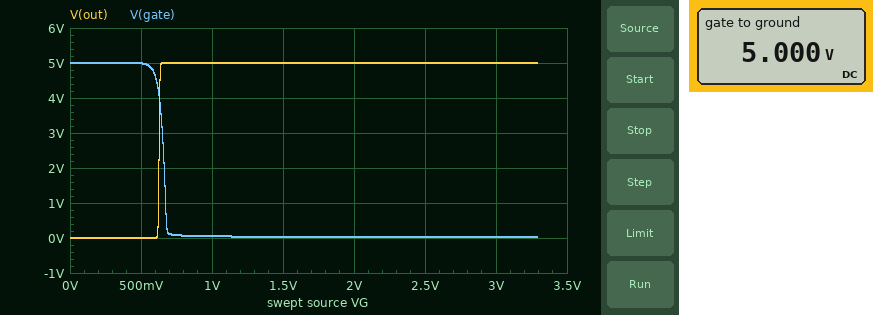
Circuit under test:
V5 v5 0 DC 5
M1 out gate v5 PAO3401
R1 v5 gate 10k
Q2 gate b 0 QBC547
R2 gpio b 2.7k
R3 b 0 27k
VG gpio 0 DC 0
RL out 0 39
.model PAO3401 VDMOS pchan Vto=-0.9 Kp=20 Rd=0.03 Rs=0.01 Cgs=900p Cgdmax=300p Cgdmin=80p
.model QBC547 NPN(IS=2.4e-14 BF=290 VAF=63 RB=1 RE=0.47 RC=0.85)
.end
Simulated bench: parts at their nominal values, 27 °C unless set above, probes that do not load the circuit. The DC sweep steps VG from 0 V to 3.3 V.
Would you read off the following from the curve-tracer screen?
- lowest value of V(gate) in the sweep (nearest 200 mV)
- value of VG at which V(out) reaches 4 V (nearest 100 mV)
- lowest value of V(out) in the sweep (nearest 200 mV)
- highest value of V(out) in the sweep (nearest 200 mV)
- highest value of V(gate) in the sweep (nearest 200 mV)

0 V
600 mV
0 V
5.0 V
5.0 V
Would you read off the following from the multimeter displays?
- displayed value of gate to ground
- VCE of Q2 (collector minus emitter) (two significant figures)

5.000 V
5.0 V
